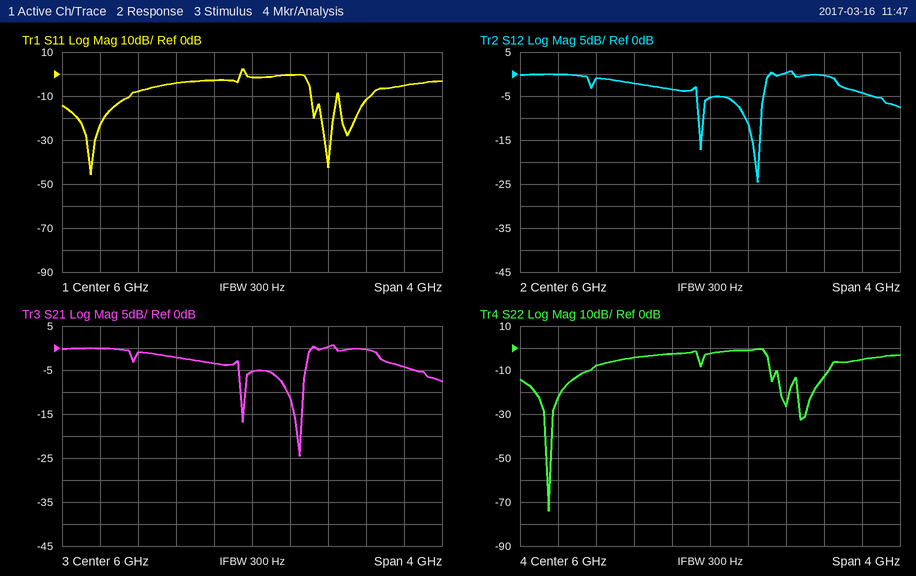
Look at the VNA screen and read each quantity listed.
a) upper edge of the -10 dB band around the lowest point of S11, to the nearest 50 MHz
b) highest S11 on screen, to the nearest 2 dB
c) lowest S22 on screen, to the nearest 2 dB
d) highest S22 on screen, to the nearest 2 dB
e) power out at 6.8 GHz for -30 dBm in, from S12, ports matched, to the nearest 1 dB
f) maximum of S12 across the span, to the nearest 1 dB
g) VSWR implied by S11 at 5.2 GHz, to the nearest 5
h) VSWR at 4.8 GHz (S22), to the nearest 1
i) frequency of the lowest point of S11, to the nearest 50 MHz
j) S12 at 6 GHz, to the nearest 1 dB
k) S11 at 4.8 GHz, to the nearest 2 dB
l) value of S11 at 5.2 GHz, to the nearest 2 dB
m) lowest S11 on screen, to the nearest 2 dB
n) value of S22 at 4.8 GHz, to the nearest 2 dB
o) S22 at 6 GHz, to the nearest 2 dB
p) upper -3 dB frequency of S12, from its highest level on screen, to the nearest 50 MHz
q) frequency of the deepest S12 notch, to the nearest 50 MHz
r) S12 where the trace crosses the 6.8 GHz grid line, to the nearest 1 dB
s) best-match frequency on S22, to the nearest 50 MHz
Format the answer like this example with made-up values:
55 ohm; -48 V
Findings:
4.70 GHz; 2 dB; -74 dB; 0 dB; -30 dBm; 1 dB; 5; 2; 4.30 GHz; -5 dB; -8 dB; -4 dB; -46 dB; -8 dB; -2 dB; 7.35 GHz; 6.50 GHz; 0 dB; 4.30 GHz
